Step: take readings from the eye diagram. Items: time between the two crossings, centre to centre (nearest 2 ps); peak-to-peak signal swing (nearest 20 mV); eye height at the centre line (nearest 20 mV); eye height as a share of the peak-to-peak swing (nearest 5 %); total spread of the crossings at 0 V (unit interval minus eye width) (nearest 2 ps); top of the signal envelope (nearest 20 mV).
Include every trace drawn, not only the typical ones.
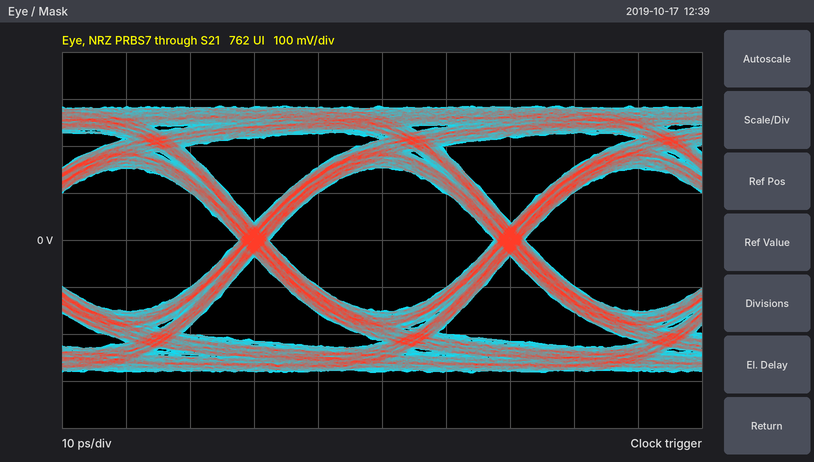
40 ps
560 mV
300 mV
55 %
4 ps
280 mV
